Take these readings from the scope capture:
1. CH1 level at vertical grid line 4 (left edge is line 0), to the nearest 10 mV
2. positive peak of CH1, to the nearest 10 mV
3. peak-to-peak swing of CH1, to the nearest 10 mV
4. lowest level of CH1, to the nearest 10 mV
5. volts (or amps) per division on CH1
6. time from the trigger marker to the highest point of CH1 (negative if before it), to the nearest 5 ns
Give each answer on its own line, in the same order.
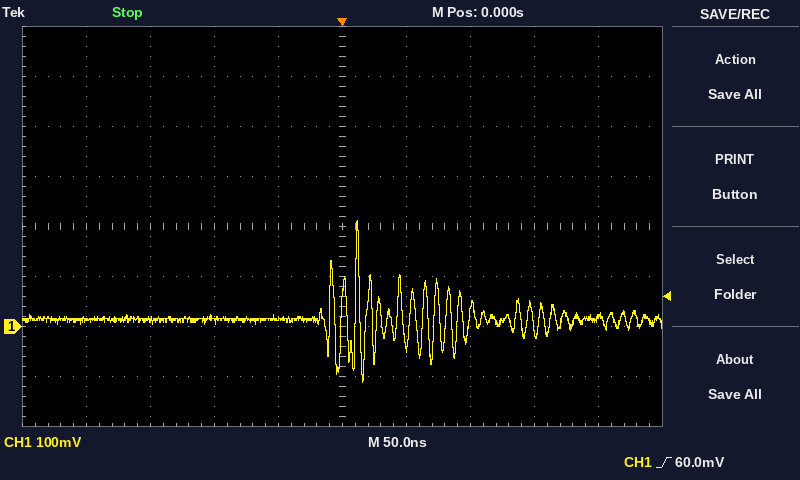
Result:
20 mV
210 mV
320 mV
-110 mV
100 mV
+10 ns
